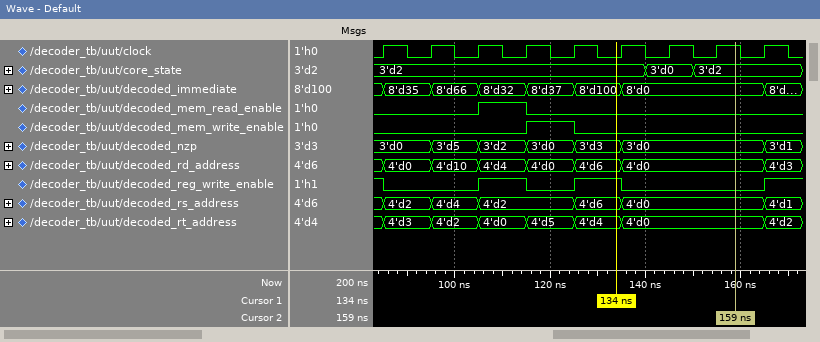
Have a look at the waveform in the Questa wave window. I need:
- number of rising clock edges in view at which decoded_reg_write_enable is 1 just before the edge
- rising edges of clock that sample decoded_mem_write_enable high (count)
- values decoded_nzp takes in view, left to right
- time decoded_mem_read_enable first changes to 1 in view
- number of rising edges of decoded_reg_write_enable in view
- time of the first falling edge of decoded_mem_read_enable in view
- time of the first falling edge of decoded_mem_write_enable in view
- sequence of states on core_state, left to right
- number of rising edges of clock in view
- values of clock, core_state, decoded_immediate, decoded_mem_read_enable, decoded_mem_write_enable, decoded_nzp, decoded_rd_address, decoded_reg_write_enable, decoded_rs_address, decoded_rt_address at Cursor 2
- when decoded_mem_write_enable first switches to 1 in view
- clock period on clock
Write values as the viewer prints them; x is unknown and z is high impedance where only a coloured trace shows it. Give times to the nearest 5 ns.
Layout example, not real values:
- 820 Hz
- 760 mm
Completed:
- 3
- 1
- 3'd0, 3'd5, 3'd2, 3'd0, 3'd3, 3'd0, 3'd1
- 105 ns
- 3
- 115 ns
- 125 ns
- 3'd2, 3'd0, 3'd2
- 9
- clock=1, core_state=3'd2, decoded_immediate=8'd0, decoded_mem_read_enable=0, decoded_mem_write_enable=0, decoded_nzp=3'd0, decoded_rd_address=4'd0, decoded_reg_write_enable=0, decoded_rs_address=4'd0, decoded_rt_address=4'd0
- 115 ns
- 10 ns
